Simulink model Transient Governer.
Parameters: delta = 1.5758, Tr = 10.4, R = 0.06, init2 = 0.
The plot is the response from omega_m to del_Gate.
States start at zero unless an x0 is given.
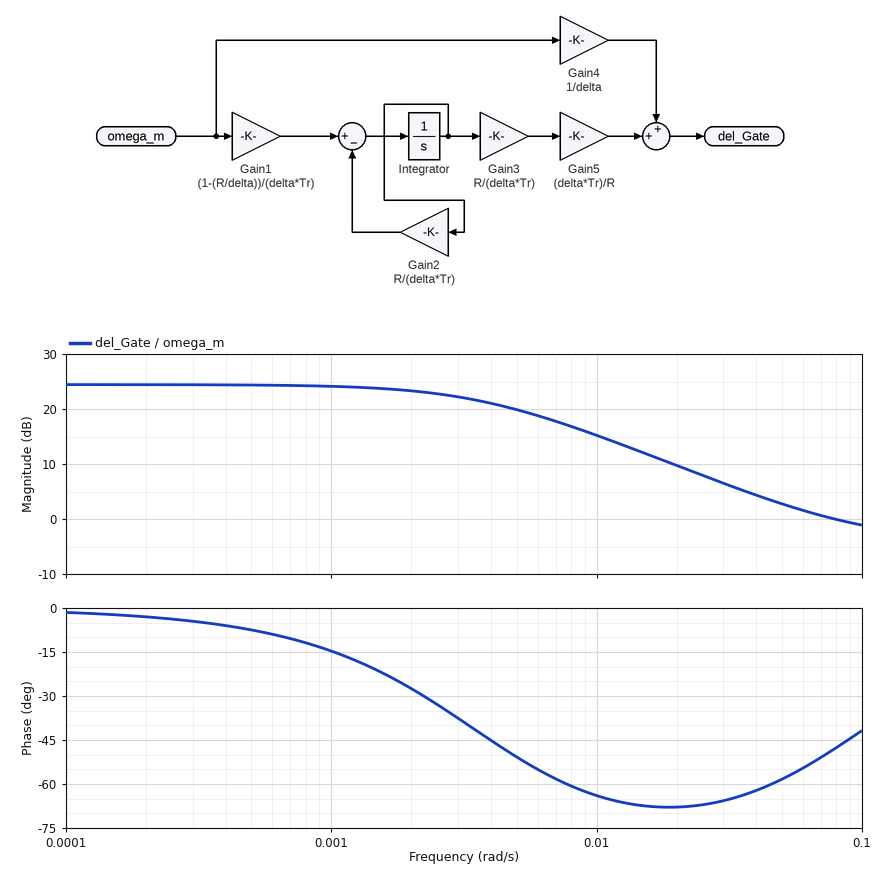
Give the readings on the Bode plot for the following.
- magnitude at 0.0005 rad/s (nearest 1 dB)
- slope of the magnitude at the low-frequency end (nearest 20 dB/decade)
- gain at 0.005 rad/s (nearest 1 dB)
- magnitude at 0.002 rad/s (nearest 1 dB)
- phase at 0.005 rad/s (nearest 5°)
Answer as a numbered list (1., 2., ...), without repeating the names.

1. 24 dB
2. 0 dB/decade
3. 20 dB
4. 23 dB
5. -50°
